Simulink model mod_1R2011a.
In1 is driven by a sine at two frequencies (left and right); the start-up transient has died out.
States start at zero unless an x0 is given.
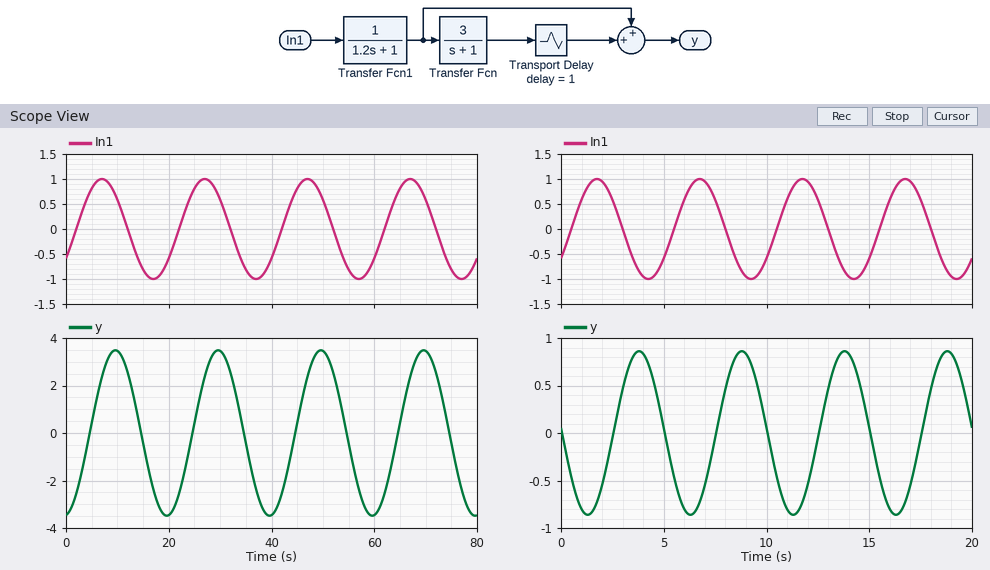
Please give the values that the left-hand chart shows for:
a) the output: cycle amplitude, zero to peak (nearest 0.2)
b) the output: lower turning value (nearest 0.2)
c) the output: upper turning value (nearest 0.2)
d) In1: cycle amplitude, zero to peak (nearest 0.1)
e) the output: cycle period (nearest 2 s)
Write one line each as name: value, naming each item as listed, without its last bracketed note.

the output: cycle amplitude, zero to peak: 3.4
the output: lower turning value: -3.4
the output: upper turning value: 3.4
In1: cycle amplitude, zero to peak: 1.0
the output: cycle period: 20 s
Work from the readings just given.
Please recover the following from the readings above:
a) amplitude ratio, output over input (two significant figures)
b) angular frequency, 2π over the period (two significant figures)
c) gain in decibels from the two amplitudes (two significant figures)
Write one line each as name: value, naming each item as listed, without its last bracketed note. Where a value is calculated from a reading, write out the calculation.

amplitude ratio, output over input: 3.4 / 1 = 3.4
angular frequency, 2π over the period: 2π / 20 = 0.31 rad/s
gain in decibels from the two amplitudes: 20 log10(3.4 / 1) = 11 dB
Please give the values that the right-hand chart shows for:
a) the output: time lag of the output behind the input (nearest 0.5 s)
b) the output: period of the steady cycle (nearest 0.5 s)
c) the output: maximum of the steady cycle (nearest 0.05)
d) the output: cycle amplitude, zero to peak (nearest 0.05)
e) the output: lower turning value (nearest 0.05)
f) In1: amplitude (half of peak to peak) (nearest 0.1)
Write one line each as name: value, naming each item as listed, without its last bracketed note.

the output: time lag of the output behind the input: 2.0 s
the output: period of the steady cycle: 5.0 s
the output: maximum of the steady cycle: 0.85
the output: cycle amplitude, zero to peak: 0.85
the output: lower turning value: -0.85
In1: amplitude (half of peak to peak): 1.0
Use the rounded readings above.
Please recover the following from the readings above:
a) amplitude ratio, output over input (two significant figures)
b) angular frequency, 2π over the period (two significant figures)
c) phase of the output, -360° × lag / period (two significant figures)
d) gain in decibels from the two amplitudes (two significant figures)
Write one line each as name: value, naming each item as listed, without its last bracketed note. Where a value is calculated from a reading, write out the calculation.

amplitude ratio, output over input: 0.85 / 1 = 0.85
angular frequency, 2π over the period: 2π / 5 = 1.3 rad/s
phase of the output, -360° × lag / period: -360 × 2 / 5 = -140°
gain in decibels from the two amplitudes: 20 log10(0.85 / 1) = -1.4 dB
